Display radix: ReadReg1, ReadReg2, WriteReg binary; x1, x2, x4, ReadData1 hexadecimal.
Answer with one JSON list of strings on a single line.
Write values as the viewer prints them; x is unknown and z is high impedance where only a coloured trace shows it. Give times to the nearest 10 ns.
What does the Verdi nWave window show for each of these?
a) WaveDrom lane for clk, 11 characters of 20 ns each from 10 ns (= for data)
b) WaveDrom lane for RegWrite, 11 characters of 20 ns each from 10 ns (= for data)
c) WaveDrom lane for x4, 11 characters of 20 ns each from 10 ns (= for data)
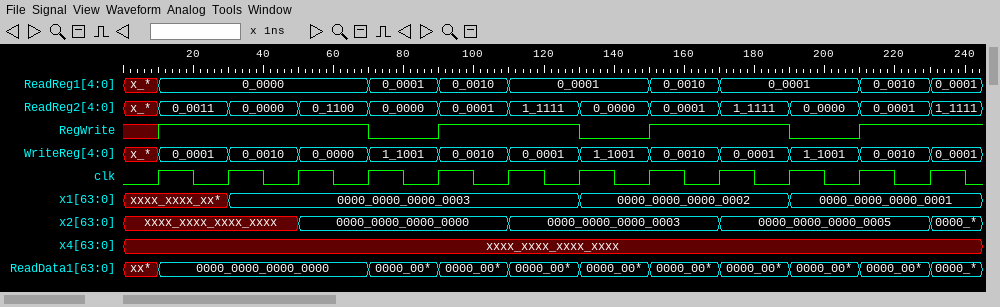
["{name: 'clk', wave: 'p..........'}", "{name: 'RegWrite', wave: '1..01.01.01'}", "{name: 'x4', wave: 'x..........'}"]
